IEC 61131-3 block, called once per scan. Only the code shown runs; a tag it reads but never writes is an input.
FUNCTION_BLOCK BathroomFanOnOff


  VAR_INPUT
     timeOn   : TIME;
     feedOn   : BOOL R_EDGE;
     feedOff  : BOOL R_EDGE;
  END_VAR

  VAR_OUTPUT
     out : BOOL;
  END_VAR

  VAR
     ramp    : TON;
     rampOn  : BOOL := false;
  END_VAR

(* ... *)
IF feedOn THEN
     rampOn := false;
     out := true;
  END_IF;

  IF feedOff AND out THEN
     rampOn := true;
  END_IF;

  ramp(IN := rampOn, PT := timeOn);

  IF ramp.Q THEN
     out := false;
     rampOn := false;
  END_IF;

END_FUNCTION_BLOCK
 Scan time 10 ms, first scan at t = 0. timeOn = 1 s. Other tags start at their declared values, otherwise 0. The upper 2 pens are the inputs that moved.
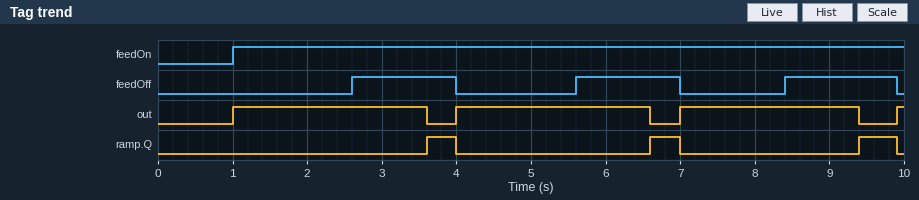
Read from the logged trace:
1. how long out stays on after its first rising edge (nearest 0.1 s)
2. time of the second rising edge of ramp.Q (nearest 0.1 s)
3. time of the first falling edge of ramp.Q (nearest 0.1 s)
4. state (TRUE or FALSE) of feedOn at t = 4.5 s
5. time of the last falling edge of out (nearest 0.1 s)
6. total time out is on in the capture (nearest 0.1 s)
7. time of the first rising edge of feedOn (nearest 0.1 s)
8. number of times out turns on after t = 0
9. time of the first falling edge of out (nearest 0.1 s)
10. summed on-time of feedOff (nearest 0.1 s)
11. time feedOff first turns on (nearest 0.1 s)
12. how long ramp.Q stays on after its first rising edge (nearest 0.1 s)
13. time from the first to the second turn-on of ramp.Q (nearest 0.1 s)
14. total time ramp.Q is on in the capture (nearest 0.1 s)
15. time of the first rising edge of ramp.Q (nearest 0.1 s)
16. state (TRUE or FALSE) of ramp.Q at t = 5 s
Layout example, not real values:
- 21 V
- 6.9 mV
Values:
- 2.6 s
- 6.6 s
- 4.0 s
- TRUE
- 9.4 s
- 7.7 s
- 1.0 s
- 4
- 3.6 s
- 4.3 s
- 2.6 s
- 0.4 s
- 3.0 s
- 1.3 s
- 3.6 s
- FALSE
